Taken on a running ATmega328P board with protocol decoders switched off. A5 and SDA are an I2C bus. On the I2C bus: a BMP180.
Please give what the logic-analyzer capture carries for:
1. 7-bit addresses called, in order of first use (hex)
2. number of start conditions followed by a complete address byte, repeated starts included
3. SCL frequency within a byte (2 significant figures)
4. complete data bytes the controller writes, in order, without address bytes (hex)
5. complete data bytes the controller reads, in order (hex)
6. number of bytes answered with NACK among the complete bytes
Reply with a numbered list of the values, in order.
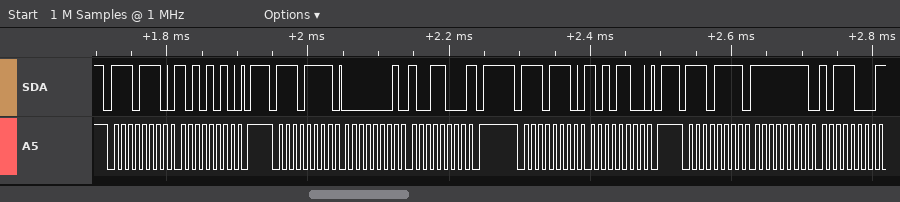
1. 0x77
2. 4
3. 100 kHz
4. AA AC
5. 01 98 FF B8
6. 2
